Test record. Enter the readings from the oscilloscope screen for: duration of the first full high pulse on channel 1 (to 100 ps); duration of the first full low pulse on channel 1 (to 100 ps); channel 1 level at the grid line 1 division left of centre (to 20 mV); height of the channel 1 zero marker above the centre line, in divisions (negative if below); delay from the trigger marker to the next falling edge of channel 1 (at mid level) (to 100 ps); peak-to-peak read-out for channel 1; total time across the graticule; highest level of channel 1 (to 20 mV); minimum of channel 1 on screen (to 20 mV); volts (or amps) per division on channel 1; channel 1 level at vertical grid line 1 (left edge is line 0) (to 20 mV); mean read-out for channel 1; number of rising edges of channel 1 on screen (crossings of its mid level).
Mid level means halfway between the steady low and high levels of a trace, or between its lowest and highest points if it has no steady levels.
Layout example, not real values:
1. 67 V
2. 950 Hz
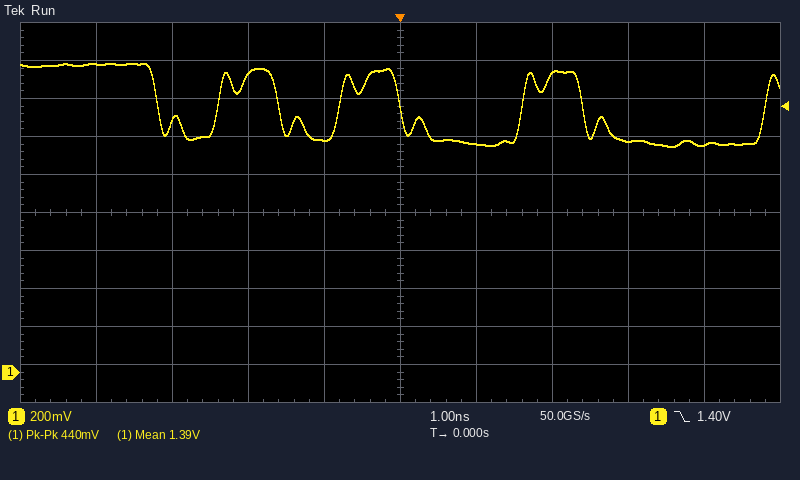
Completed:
1. 800 ps
2. 800 ps
3. 1.22 V
4. -4.2 div
5. 2.4 ns
6. 440 mV
7. 10 ns
8. 1.62 V
9. 1.18 V
10. 200 mV
11. 1.62 V
12. 1.39 V
13. 4
